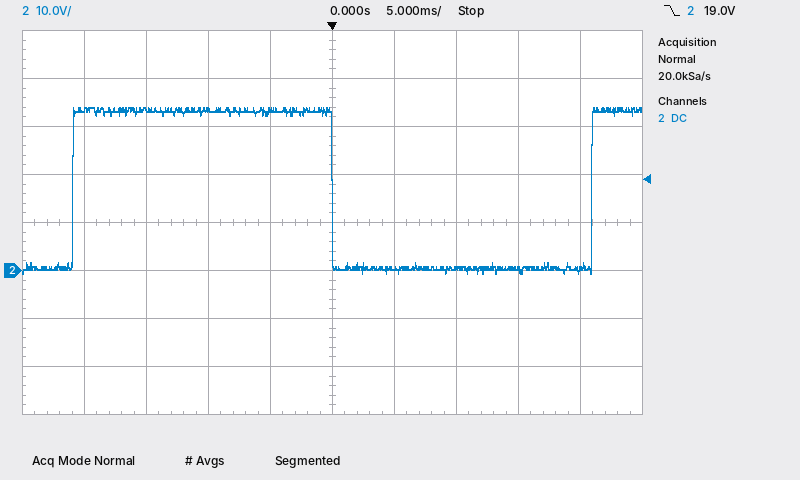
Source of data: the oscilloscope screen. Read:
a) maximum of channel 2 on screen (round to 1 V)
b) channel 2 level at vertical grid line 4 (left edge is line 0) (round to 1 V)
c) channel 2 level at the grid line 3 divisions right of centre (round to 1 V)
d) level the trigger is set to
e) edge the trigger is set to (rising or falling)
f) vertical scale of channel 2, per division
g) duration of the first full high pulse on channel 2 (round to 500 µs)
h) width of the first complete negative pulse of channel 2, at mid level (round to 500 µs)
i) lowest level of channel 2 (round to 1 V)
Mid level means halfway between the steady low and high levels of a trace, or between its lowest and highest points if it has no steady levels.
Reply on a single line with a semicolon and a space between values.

34 V; 33 V; 0 V; 19.0 V; falling; 10 V; 21.0 ms; 21.0 ms; -1 V
